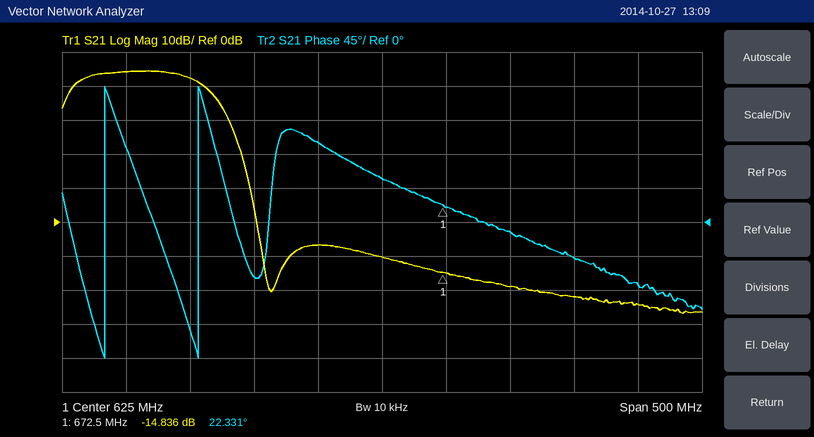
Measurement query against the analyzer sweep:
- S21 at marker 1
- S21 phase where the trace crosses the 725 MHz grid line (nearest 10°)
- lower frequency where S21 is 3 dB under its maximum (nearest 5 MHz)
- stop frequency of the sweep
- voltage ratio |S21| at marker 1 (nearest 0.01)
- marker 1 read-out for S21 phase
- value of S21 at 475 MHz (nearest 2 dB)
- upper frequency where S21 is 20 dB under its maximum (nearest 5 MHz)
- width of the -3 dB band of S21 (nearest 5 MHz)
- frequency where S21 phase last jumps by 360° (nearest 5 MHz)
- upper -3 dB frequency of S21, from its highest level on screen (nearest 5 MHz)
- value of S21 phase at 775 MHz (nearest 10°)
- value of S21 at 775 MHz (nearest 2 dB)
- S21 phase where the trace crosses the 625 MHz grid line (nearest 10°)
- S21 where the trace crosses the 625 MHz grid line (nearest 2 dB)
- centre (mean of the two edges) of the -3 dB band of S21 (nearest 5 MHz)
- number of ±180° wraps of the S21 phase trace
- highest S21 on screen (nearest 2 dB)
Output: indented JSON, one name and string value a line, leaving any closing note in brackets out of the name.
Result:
{
  "S21 at marker 1": "-14.836 dB",
  "S21 phase where the trace crosses the 725 MHz grid line": "-10°",
  "lower frequency where S21 is 3 dB under its maximum": "390 MHz",
  "stop frequency of the sweep": "875 MHz",
  "voltage ratio |S21| at marker 1": "0.18",
  "marker 1 read-out for S21 phase": "22.331°",
  "value of S21 at 475 MHz": "42 dB",
  "upper frequency where S21 is 20 dB under its maximum": "510 MHz",
  "width of the -3 dB band of S21": "90 MHz",
  "frequency where S21 phase last jumps by 360°": "480 MHz",
  "upper -3 dB frequency of S21, from its highest level on screen": "480 MHz",
  "value of S21 phase at 775 MHz": "-50°",
  "value of S21 at 775 MHz": "-22 dB",
  "S21 phase where the trace crosses the 625 MHz grid line": "60°",
  "S21 where the trace crosses the 625 MHz grid line": "-10 dB",
  "centre (mean of the two edges) of the -3 dB band of S21": "435 MHz",
  "number of ±180° wraps of the S21 phase trace": "2",
  "highest S21 on screen": "44 dB"
}
